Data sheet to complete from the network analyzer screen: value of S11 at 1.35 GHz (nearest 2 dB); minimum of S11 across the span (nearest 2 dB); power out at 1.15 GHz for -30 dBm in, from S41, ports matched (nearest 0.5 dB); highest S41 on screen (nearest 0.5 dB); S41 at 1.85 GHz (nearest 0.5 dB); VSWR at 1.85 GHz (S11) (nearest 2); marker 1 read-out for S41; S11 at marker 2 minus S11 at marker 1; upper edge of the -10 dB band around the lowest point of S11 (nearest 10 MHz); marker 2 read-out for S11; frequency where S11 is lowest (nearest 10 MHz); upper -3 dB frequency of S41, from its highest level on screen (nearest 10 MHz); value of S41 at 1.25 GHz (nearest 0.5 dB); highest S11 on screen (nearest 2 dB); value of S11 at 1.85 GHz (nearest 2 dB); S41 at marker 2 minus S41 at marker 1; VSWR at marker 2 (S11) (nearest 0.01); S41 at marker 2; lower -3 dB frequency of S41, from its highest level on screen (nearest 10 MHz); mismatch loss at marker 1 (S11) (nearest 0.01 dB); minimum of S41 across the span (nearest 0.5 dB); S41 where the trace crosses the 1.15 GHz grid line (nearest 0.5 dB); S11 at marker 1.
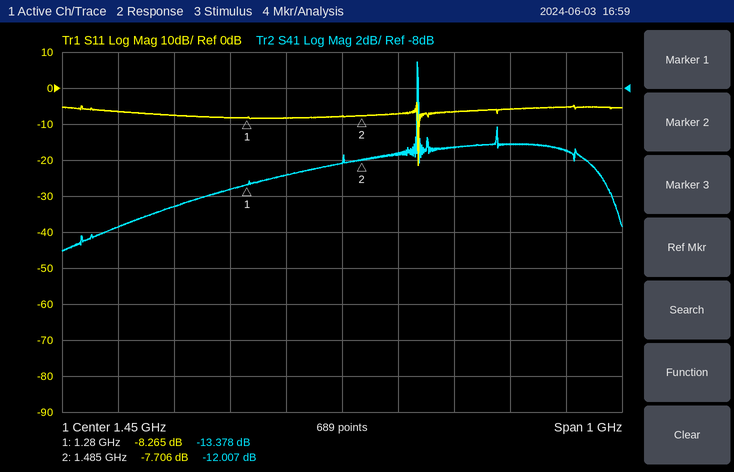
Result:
-8 dB
-22 dB
-44.5 dBm
-6.5 dB
-11.5 dB
4
-13.378 dB
0.559 dB
1.59 GHz
-7.706 dB
1.59 GHz
1.59 GHz
-13.5 dB
-4 dB
-6 dB
1.371 dB
2.40
-12.007 dB
1.58 GHz
0.70 dB
-17.0 dB
-14.5 dB
-8.265 dB
